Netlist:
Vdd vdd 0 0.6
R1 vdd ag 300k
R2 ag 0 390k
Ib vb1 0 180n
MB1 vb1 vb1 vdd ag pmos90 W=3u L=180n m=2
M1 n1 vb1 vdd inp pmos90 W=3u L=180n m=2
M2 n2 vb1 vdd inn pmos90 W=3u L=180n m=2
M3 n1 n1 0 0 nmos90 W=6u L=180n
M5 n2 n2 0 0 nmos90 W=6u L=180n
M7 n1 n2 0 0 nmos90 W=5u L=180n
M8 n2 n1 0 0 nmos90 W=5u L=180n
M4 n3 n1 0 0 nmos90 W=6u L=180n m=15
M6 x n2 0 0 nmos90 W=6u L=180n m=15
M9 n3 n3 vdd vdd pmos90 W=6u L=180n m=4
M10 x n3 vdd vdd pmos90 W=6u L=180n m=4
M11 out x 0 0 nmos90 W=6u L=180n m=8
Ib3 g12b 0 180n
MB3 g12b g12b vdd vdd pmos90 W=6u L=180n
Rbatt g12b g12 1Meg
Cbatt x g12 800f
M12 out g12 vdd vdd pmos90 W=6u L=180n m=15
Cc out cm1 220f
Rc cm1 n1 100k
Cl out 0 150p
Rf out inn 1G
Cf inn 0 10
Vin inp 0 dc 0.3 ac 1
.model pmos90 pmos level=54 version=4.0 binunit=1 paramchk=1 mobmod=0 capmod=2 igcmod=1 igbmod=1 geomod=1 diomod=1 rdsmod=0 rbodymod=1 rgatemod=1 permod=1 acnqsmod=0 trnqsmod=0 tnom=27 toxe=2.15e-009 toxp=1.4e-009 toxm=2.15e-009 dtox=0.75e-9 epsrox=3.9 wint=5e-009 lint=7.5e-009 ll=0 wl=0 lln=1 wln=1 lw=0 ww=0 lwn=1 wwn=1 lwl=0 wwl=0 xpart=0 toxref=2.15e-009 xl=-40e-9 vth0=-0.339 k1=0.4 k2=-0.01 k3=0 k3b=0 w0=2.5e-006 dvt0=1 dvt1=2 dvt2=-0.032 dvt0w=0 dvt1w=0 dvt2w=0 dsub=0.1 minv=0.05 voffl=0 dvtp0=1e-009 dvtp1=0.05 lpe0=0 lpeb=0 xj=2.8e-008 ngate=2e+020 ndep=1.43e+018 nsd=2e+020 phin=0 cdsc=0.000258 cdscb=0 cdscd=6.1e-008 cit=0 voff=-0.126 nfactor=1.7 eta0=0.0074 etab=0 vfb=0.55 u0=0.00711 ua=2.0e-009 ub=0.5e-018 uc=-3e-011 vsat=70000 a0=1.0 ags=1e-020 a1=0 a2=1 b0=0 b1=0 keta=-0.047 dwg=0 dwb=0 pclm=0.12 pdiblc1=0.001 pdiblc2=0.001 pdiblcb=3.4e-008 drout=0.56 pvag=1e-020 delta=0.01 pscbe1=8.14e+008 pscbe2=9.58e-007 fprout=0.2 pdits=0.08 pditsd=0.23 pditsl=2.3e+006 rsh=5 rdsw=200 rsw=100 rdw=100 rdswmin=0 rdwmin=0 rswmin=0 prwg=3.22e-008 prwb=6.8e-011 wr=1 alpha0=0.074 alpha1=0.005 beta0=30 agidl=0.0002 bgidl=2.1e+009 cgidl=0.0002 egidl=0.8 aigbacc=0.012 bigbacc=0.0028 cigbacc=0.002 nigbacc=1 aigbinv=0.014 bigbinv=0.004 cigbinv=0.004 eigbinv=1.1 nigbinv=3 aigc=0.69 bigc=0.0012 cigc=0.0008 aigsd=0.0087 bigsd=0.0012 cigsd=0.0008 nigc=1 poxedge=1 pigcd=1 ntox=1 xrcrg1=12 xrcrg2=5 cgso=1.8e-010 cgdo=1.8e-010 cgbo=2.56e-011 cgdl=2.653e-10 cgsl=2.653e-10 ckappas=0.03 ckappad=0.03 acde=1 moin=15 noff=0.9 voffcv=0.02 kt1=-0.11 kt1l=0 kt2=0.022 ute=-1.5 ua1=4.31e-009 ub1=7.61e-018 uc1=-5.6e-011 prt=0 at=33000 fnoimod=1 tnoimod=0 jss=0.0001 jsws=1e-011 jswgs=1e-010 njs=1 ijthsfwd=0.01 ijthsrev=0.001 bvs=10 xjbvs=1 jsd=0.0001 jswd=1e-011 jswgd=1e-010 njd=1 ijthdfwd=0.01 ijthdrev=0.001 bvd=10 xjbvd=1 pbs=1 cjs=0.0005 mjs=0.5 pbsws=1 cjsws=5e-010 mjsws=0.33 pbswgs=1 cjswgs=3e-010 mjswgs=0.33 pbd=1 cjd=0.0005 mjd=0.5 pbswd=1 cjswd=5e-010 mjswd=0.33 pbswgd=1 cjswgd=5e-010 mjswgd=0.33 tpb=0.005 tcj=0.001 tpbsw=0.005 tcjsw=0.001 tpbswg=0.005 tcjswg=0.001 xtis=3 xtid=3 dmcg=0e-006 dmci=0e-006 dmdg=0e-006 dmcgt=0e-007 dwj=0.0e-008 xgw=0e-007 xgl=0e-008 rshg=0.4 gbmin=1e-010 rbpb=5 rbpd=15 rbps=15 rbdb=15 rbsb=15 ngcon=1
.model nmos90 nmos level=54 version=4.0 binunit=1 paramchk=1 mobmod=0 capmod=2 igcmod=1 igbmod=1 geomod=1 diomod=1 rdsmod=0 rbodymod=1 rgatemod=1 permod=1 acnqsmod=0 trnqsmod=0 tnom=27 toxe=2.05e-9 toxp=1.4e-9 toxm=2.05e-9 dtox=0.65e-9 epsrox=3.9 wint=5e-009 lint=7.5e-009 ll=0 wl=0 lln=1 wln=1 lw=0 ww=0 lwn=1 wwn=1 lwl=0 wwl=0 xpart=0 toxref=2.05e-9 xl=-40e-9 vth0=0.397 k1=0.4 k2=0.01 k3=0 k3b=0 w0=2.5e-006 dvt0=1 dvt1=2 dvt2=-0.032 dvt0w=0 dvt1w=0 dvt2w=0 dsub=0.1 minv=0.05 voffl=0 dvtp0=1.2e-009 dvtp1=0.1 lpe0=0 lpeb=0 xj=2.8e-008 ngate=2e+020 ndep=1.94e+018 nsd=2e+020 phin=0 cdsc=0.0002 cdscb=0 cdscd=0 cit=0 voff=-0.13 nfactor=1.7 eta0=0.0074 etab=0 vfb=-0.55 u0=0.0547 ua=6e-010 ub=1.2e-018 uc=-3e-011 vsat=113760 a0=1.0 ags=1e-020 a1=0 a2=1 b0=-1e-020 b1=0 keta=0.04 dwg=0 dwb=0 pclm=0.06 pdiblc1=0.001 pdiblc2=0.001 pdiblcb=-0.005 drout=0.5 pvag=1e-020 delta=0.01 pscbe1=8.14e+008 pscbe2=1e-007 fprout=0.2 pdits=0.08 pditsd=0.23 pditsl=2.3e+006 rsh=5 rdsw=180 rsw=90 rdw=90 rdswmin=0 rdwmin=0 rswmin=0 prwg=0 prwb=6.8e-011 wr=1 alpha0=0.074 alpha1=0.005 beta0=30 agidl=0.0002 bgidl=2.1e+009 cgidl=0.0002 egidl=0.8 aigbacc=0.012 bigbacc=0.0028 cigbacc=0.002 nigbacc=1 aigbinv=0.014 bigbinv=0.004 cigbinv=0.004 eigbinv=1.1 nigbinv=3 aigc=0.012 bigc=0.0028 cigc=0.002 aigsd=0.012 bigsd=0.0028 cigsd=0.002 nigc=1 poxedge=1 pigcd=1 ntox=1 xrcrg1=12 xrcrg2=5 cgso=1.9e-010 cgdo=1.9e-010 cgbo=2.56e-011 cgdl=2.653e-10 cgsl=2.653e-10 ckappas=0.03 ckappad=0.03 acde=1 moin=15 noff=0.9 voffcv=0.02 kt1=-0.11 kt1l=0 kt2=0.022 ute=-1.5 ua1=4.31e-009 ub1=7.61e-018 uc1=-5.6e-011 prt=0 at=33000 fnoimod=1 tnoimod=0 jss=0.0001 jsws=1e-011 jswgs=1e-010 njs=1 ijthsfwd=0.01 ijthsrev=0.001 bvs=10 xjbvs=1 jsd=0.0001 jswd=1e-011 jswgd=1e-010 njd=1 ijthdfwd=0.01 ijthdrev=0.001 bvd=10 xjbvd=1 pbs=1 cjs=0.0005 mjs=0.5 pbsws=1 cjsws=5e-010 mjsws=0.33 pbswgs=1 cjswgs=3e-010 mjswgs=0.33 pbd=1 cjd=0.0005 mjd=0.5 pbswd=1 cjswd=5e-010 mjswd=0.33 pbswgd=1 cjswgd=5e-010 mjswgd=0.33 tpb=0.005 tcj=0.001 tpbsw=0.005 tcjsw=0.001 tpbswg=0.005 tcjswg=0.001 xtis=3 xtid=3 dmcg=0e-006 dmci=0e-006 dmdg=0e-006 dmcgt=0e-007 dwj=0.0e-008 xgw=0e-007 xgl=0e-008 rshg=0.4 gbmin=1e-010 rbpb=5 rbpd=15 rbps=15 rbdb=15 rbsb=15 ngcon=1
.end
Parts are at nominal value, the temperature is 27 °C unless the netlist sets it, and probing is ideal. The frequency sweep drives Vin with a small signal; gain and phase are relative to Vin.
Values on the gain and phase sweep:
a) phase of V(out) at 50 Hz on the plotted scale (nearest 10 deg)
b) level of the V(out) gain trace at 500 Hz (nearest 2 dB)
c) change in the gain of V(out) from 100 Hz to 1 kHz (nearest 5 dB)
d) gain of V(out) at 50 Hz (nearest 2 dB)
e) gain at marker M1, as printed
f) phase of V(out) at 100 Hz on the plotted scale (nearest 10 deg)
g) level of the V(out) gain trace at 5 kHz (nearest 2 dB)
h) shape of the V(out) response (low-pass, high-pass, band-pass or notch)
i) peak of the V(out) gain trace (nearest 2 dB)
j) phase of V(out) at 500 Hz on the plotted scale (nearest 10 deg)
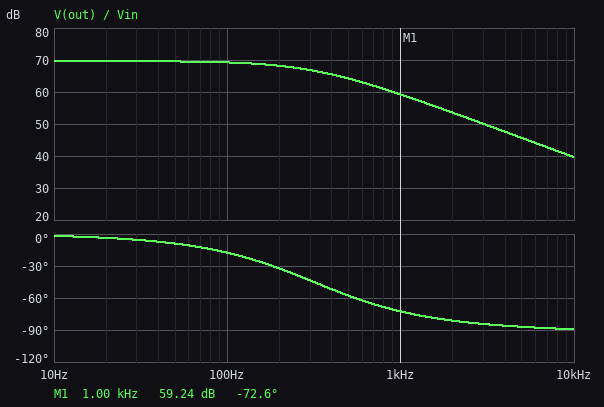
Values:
-10 deg
64 dB
-10 dB
70 dB
59.24 dB
-20 deg
46 dB
low-pass
70 dB
-60 deg
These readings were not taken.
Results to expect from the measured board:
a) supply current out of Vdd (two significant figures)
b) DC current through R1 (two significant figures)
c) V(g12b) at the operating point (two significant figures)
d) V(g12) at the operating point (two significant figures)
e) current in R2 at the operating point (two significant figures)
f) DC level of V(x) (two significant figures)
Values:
9.1 µA
870 nA
410 mV
410 mV
870 nA
170 mV
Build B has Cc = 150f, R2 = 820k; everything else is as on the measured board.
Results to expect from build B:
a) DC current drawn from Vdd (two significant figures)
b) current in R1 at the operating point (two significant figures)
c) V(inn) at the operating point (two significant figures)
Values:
12 µA
540 nA
300 mV
